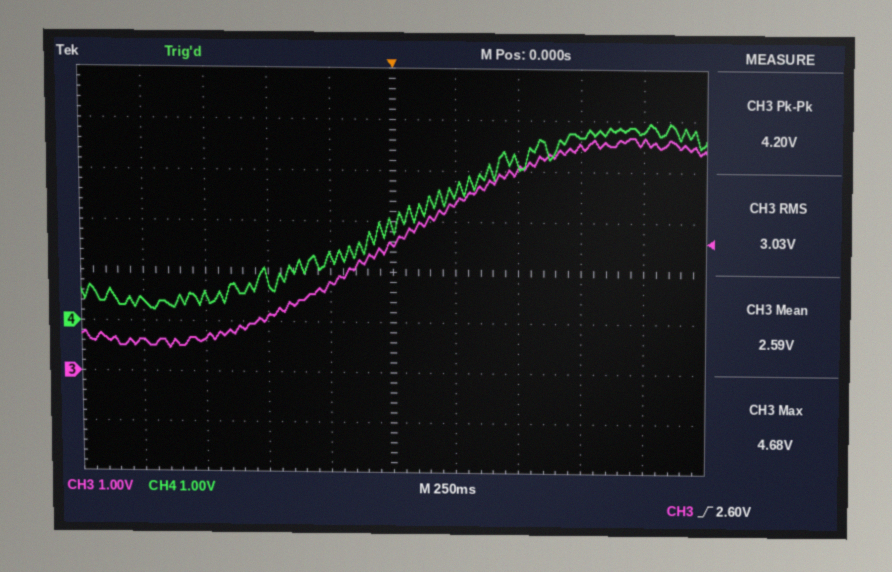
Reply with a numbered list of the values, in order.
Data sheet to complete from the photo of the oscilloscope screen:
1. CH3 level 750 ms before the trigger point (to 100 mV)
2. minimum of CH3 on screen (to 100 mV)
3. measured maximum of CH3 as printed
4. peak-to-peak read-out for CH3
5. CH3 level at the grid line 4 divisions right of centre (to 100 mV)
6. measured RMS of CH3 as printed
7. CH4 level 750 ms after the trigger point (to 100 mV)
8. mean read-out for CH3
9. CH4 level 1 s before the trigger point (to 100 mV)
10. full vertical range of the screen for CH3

1. 700 mV
2. 500 mV
3. 4.68 V
4. 4.20 V
5. 4.6 V
6. 3.03 V
7. 3.7 V
8. 2.59 V
9. 400 mV
10. 8 V
